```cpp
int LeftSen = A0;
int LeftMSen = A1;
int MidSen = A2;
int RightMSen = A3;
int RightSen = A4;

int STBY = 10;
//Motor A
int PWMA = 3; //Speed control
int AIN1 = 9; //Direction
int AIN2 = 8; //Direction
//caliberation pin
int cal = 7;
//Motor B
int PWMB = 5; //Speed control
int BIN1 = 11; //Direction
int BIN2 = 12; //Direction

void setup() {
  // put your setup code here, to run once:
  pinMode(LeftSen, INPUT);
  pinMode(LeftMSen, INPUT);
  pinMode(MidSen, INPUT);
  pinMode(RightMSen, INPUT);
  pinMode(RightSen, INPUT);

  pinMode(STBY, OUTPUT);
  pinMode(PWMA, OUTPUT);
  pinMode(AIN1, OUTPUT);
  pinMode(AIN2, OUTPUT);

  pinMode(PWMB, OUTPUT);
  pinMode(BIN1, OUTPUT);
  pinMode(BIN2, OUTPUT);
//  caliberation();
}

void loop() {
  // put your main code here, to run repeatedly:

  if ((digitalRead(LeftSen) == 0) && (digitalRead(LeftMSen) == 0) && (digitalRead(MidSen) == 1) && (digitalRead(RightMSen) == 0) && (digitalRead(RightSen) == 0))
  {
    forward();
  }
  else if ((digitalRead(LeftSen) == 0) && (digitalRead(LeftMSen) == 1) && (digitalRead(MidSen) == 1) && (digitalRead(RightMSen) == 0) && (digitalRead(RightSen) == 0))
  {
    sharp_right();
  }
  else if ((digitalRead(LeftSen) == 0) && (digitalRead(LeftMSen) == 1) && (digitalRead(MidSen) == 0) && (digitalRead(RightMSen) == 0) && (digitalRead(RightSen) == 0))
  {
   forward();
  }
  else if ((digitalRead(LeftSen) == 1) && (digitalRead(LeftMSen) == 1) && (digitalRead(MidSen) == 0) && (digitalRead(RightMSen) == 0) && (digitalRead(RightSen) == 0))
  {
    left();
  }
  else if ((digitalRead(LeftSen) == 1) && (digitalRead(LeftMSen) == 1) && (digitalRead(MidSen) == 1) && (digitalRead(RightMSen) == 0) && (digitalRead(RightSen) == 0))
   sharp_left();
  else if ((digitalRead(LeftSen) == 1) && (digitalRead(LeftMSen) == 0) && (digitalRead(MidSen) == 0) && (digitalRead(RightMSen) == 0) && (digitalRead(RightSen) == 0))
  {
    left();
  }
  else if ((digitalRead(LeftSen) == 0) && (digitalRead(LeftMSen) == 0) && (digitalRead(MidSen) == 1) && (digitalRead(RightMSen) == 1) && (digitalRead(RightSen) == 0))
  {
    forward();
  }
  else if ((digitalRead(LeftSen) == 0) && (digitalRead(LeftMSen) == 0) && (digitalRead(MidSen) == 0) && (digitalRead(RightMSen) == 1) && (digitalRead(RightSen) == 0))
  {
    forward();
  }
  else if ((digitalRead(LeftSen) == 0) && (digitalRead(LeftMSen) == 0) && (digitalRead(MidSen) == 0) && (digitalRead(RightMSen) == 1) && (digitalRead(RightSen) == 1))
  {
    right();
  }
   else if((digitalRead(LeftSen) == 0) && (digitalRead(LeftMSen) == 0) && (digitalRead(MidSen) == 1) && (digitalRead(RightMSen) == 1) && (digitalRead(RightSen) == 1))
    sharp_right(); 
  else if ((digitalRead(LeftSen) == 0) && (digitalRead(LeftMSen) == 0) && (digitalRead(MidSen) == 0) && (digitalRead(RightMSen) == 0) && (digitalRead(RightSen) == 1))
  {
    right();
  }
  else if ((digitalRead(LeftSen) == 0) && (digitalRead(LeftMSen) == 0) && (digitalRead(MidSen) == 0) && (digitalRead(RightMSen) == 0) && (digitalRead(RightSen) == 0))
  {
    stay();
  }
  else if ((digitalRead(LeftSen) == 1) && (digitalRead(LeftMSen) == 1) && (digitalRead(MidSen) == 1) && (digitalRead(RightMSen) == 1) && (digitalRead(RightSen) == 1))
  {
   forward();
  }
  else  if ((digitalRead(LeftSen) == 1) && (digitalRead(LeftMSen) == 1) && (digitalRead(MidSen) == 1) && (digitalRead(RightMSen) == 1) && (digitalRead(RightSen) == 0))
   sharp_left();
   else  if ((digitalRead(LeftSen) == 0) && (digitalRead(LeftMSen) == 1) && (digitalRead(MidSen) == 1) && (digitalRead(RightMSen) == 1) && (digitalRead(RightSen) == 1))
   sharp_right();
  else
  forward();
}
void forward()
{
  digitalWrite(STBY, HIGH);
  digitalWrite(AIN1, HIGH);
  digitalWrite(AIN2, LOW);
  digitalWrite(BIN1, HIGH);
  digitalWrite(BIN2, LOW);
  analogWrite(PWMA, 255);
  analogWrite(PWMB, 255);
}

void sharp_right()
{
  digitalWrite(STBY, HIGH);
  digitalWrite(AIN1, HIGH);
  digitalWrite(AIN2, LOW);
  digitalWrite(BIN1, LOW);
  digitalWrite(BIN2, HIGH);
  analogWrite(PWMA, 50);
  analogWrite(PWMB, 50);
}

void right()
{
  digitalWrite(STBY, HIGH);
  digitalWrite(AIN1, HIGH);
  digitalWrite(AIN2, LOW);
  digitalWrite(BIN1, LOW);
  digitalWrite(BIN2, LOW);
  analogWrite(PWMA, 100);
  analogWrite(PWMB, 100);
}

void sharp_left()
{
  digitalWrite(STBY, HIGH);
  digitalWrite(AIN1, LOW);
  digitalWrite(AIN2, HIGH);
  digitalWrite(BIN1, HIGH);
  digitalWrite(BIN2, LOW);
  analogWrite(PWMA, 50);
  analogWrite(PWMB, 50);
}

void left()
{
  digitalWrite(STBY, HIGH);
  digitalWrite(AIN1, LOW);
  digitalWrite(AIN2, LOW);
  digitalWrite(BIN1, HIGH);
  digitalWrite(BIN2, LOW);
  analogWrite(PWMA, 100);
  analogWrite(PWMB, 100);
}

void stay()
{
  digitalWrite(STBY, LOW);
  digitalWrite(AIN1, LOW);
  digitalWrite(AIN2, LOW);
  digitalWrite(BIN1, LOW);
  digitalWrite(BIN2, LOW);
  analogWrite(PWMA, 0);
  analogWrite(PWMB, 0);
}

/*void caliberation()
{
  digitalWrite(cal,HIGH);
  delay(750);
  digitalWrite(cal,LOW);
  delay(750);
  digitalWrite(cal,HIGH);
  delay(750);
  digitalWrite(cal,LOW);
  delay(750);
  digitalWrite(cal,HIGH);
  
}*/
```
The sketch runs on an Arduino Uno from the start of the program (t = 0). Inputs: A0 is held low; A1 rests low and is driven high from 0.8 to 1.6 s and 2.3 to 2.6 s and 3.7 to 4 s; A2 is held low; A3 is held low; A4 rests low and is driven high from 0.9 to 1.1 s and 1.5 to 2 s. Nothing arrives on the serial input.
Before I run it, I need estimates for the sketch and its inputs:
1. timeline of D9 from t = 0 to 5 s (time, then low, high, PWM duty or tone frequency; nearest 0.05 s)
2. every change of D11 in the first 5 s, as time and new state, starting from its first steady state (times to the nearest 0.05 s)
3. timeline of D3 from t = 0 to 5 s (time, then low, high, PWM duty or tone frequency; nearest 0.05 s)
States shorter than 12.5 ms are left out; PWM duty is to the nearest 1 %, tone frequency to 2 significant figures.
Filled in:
0 s low; 0.8 s high; 2 s low; 2.3 s high; 2.6 s low; 3.7 s high; 4 s low
0 s low; 0.8 s high; 1.6 s low; 2.3 s high; 2.6 s low; 3.7 s high; 4 s low
0 s low; 0.8 s high; 1.6 s PWM 39 %; 2 s low; 2.3 s high; 2.6 s low; 3.7 s high; 4 s low
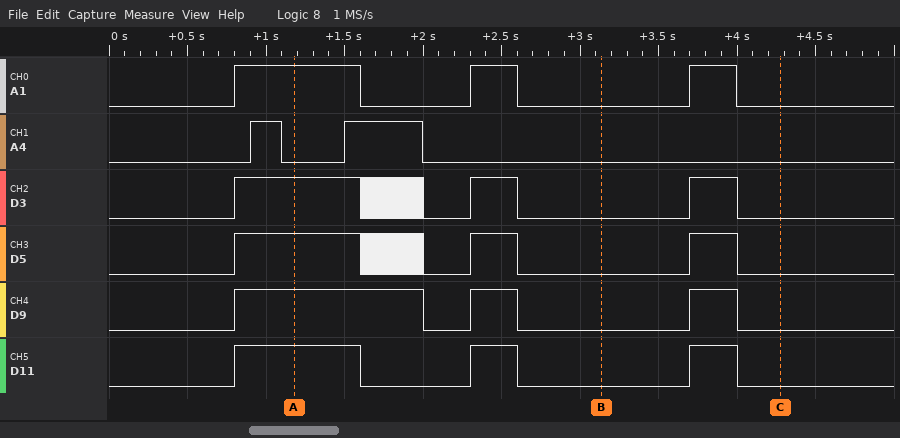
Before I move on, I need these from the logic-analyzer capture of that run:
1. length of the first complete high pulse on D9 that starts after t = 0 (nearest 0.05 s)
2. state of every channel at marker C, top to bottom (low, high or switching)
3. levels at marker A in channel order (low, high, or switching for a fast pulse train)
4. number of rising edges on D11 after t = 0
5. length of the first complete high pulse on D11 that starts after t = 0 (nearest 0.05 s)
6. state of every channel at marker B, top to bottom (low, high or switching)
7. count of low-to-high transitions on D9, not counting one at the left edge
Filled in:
1.20 s
A1 low, A4 low, D3 low, D5 low, D9 low, D11 low
A1 high, A4 low, D3 high, D5 high, D9 high, D11 high
3
0.80 s
A1 low, A4 low, D3 low, D5 low, D9 low, D11 low
3
